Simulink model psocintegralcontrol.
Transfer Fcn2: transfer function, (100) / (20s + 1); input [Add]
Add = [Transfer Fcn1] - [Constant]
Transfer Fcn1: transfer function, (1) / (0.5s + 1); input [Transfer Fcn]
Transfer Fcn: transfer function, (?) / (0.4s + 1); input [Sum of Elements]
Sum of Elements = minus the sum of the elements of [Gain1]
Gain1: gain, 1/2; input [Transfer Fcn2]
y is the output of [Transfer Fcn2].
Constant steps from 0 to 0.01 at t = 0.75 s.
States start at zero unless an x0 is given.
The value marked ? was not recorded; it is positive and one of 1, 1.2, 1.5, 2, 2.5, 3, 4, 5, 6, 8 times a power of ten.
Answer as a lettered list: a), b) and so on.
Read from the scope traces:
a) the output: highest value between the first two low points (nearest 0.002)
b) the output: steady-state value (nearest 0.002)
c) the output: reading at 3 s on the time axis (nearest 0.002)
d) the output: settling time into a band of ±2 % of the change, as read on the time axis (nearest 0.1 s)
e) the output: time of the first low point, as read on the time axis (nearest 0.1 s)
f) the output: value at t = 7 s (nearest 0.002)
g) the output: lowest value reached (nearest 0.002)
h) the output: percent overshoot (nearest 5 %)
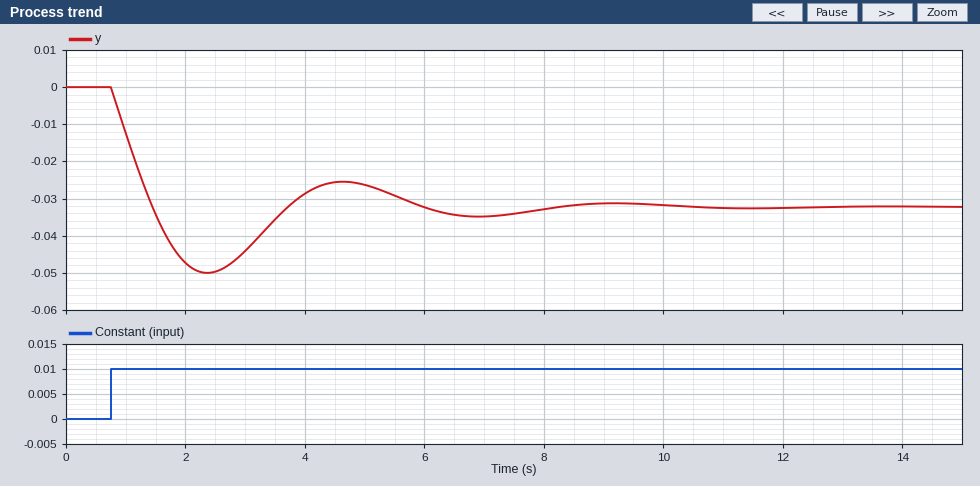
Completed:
a) -0.026
b) -0.032
c) -0.044
d) 9.8 s
e) 2.4 s
f) -0.034
g) -0.050
h) 55 %
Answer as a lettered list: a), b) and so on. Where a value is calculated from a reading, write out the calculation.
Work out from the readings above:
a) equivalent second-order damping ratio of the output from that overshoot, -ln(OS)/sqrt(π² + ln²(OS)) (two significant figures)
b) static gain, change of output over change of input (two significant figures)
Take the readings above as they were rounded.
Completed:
a) ln(0.55) = -0.598; 0.598 / sqrt(9.870 + 0.357) = 0.19
b) (-0.032 - 0) / (0.01 - 0) = -3.2
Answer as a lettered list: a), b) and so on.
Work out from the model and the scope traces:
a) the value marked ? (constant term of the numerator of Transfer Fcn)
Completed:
a) 0.6
